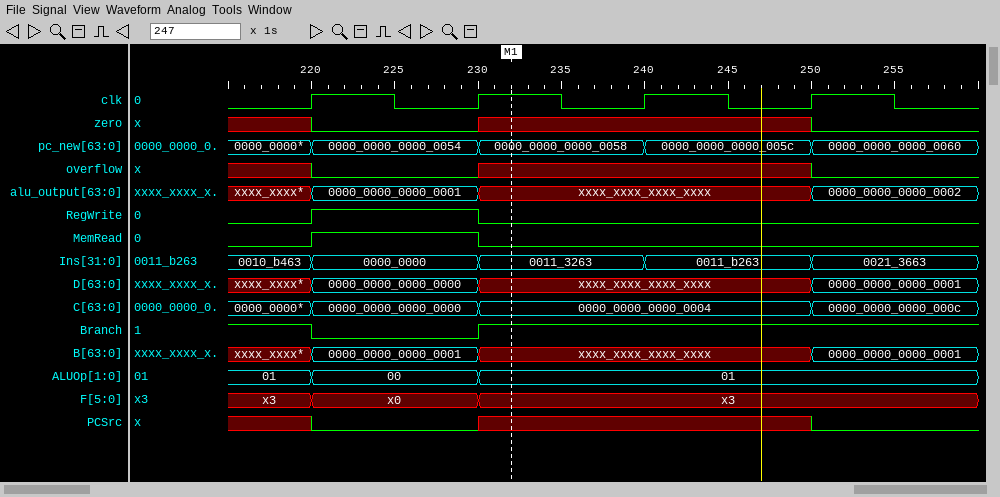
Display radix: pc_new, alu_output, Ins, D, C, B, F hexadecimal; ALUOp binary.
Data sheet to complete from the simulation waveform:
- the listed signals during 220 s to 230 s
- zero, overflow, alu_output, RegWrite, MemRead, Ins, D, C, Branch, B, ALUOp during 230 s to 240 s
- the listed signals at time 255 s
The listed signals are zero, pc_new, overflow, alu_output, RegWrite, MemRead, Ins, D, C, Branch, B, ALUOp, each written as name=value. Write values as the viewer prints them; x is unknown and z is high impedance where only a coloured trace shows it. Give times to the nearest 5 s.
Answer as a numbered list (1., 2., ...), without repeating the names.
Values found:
1. zero=0, pc_new=0000_0000_0000_0054, overflow=0, alu_output=0000_0000_0000_0001, RegWrite=1, MemRead=1, Ins=0000_0000, D=0000_0000_0000_0000, C=0000_0000_0000_0000, Branch=0, B=0000_0000_0000_0001, ALUOp=00
2. zero=x, overflow=x, alu_output=xxxx_xxxx_xxxx_xxxx, RegWrite=0, MemRead=0, Ins=0011_3263, D=xxxx_xxxx_xxxx_xxxx, C=0000_0000_0000_0004, Branch=1, B=xxxx_xxxx_xxxx_xxxx, ALUOp=01
3. zero=0, pc_new=0000_0000_0000_0060, overflow=0, alu_output=0000_0000_0000_0002, RegWrite=0, MemRead=0, Ins=0021_3663, D=0000_0000_0000_0001, C=0000_0000_0000_000c, Branch=1, B=0000_0000_0000_0001, ALUOp=01
